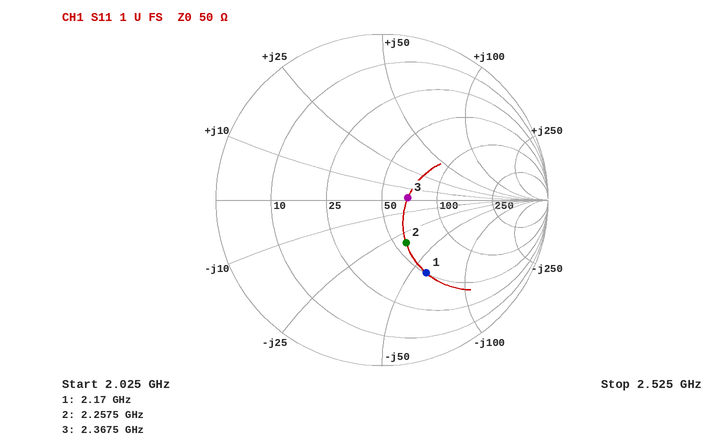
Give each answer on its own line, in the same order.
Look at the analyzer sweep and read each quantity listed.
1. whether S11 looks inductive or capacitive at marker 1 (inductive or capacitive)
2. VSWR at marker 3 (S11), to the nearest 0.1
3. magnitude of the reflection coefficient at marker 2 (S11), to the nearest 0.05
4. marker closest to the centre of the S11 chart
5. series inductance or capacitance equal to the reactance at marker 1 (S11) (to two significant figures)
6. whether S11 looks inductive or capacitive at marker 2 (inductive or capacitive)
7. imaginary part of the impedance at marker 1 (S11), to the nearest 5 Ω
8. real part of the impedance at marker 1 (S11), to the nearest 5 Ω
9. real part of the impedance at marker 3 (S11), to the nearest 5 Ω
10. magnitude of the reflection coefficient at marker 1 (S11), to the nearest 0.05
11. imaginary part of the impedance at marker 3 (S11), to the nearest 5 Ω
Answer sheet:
capacitive
1.4
0.30
marker 3
1.2 pF
capacitive
-60 Ω
50 Ω
70 Ω
0.50
0 Ω
